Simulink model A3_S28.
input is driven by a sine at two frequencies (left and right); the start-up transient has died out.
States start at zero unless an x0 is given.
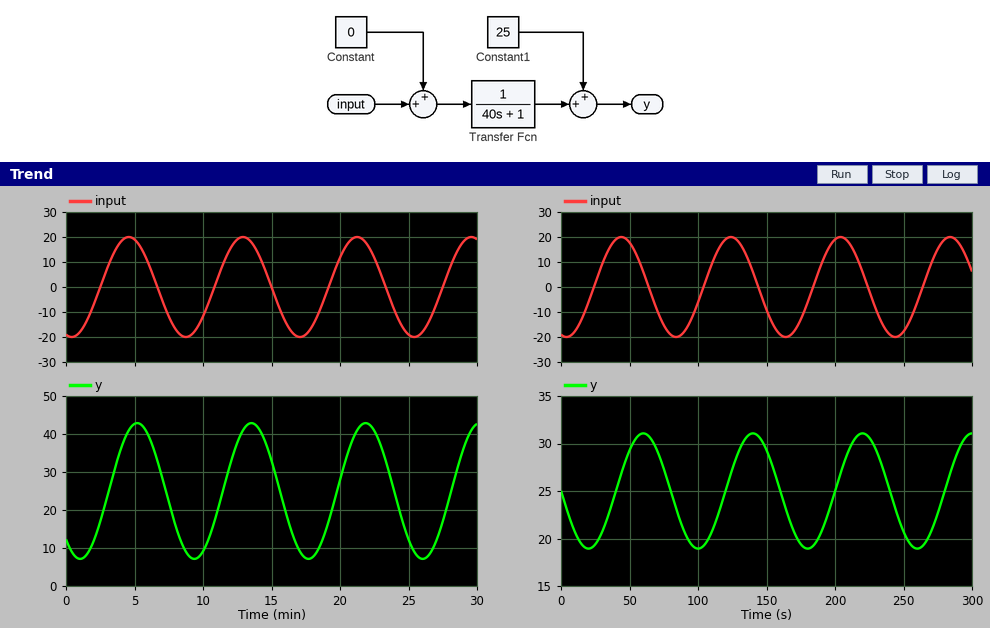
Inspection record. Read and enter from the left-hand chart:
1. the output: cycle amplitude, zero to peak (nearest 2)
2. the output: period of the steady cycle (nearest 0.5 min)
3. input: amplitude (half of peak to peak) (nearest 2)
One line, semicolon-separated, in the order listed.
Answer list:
18; 8.5 min; 20
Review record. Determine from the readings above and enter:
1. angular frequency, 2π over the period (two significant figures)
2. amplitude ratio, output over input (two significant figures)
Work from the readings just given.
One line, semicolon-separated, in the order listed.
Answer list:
0.74 rad/min; 0.90
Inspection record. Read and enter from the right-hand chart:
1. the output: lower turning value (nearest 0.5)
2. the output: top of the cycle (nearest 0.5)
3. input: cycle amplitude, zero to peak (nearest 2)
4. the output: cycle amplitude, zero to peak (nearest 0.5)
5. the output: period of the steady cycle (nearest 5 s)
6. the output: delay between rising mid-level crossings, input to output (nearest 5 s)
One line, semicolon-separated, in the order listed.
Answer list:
19.0; 31.0; 20; 6.0; 80 s; 15 s
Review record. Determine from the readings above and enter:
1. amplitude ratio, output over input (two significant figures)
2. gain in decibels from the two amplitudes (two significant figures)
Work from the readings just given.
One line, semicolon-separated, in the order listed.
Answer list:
0.30; -10 dB
